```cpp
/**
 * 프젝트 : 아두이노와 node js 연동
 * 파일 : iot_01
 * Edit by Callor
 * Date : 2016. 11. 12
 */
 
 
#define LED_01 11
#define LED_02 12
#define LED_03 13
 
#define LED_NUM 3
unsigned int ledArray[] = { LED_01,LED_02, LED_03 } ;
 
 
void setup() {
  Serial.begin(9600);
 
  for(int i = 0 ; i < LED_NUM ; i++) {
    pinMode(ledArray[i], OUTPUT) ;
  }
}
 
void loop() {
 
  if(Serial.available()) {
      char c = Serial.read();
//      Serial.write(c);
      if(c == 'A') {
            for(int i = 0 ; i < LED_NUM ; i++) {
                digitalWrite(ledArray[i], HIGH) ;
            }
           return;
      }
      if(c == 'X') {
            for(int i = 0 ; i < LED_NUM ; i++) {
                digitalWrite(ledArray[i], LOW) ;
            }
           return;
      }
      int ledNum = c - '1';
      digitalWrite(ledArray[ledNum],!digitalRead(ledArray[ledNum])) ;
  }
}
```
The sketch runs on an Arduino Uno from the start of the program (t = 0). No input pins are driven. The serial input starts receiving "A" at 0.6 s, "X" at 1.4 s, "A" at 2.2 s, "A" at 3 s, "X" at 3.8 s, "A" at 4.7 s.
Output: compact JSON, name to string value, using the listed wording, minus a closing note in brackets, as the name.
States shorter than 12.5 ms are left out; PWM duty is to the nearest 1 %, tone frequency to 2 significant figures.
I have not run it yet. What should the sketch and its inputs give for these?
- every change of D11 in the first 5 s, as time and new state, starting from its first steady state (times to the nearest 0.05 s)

{"every change of D11 in the first 5 s, as time and new state, starting from its first steady state": "0 s low; 0.6 s high; 1.4 s low; 2.2 s high; 3.8 s low; 4.7 s high"}
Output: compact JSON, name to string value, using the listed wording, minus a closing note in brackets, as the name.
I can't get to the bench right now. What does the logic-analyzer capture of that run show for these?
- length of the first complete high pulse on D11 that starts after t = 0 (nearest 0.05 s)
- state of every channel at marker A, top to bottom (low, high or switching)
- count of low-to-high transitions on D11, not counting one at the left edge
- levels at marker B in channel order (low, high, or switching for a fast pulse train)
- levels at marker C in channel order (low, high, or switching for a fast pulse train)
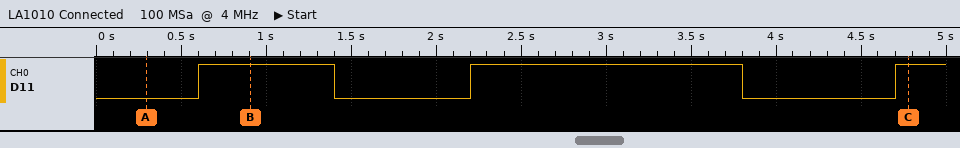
{"length of the first complete high pulse on D11 that starts after t = 0": "0.80 s", "state of every channel at marker A, top to bottom": "D11 low", "count of low-to-high transitions on D11, not counting one at the left edge": "3", "levels at marker B in channel order": "D11 high", "levels at marker C in channel order": "D11 high"}
